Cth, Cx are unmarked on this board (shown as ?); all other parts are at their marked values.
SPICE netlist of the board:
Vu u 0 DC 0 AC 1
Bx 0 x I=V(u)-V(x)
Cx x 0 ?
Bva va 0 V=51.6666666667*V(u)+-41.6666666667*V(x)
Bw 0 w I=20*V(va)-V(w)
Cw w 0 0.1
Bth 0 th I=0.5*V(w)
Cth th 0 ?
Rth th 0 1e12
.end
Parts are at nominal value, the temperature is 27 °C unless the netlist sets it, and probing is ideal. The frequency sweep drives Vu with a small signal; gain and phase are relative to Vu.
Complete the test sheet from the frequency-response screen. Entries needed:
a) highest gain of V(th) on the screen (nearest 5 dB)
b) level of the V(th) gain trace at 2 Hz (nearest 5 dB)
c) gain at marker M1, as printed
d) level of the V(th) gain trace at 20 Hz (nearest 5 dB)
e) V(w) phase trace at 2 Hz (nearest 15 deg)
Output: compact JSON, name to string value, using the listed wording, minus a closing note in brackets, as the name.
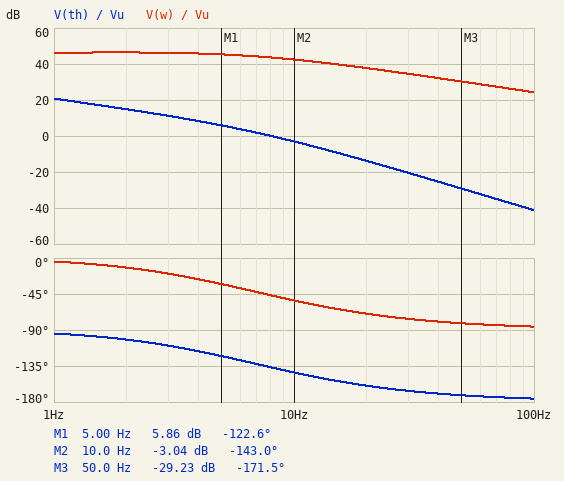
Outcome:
{"highest gain of V(th) on the screen": "20 dB", "level of the V(th) gain trace at 2 Hz": "15 dB", "gain at marker M1, as printed": "5.86 dB", "level of the V(th) gain trace at 20 Hz": "-15 dB", "V(w) phase trace at 2 Hz": "-15 deg"}
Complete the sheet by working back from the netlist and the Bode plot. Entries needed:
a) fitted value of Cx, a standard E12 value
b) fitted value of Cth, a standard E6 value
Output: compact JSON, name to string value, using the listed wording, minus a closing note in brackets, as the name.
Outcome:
{"fitted value of Cx, a standard E12 value": "22 mF", "fitted value of Cth, a standard E6 value": "1.5 F"}
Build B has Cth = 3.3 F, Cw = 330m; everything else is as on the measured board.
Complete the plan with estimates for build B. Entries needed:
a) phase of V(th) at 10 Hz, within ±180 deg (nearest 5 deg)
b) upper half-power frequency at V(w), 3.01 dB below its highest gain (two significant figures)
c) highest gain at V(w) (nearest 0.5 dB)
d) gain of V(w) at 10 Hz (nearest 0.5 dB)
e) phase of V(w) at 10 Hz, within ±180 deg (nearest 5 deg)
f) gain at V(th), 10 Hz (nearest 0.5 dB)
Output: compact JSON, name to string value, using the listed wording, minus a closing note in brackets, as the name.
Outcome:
{"phase of V(th) at 10 Hz, within ±180 deg": "-150 deg", "upper half-power frequency at V(w), 3.01 dB below its highest gain": "550 mHz", "highest gain at V(w)": "46.0 dB", "gain of V(w) at 10 Hz": "32.0 dB", "phase of V(w) at 10 Hz, within ±180 deg": "-60 deg", "gain at V(th), 10 Hz": "-20.0 dB"}
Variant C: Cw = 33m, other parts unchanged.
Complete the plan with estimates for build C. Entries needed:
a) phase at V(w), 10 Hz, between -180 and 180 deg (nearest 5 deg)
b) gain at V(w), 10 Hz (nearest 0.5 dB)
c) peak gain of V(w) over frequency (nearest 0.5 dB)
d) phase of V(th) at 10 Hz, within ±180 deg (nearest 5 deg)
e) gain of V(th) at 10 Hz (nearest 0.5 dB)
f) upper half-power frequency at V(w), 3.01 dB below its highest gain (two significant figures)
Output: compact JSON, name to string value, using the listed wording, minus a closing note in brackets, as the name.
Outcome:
{"phase at V(w), 10 Hz, between -180 and 180 deg": "-35 deg", "gain at V(w), 10 Hz": "51.5 dB", "peak gain of V(w) over frequency": "52.5 dB", "phase of V(th) at 10 Hz, within ±180 deg": "-125 deg", "gain of V(th) at 10 Hz": "6.0 dB", "upper half-power frequency at V(w), 3.01 dB below its highest gain": "14 Hz"}
